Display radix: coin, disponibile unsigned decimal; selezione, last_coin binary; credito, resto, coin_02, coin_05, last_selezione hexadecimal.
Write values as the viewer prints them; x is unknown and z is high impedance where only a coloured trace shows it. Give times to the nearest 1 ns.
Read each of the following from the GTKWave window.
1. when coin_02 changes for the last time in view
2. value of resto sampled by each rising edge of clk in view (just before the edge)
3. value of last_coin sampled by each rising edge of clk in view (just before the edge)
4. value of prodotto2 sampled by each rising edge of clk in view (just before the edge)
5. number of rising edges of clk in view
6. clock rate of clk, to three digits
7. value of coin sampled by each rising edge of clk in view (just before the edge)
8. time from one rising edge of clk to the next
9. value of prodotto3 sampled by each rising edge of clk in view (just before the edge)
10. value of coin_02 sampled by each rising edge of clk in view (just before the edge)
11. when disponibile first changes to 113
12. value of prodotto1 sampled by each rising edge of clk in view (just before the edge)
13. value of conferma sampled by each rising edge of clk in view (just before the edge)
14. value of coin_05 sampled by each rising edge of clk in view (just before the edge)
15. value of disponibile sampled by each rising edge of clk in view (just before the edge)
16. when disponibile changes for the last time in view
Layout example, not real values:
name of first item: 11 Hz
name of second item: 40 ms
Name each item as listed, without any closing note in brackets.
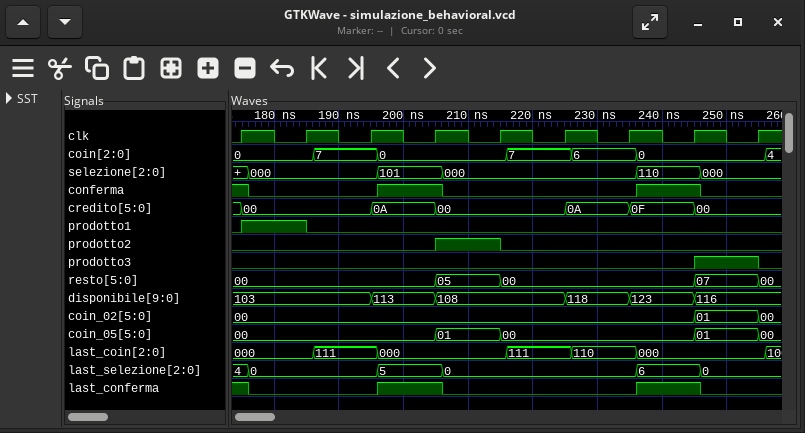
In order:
when coin_02 changes for the last time in view: 255 ns
value of resto sampled by each rising edge of clk in view: 00, 00, 00, 00, 05, 00, 00, 00, 07
value of last_coin sampled by each rising edge of clk in view: 000, 000, 111, 000, 000, 111, 110, 000, 000
value of prodotto2 sampled by each rising edge of clk in view: 0 0 0 0 1 0 0 0 0
number of rising edges of clk in view: 9
clock rate of clk, to three digits: 100 MHz
value of coin sampled by each rising edge of clk in view: 0, 0, 7, 0, 0, 7, 6, 0, 0
time from one rising edge of clk to the next: 10 ns
value of prodotto3 sampled by each rising edge of clk in view: 0 0 0 0 0 0 0 0 1
value of coin_02 sampled by each rising edge of clk in view: 00, 00, 00, 00, 00, 00, 00, 00, 01
when disponibile first changes to 113: 195 ns
value of prodotto1 sampled by each rising edge of clk in view: 0 1 0 0 0 0 0 0 0
value of conferma sampled by each rising edge of clk in view: 1 0 0 1 0 0 0 1 0
value of coin_05 sampled by each rising edge of clk in view: 00, 00, 00, 00, 01, 00, 00, 00, 01
value of disponibile sampled by each rising edge of clk in view: 103, 103, 103, 113, 108, 108, 118, 123, 116
when disponibile changes for the last time in view: 245 ns
